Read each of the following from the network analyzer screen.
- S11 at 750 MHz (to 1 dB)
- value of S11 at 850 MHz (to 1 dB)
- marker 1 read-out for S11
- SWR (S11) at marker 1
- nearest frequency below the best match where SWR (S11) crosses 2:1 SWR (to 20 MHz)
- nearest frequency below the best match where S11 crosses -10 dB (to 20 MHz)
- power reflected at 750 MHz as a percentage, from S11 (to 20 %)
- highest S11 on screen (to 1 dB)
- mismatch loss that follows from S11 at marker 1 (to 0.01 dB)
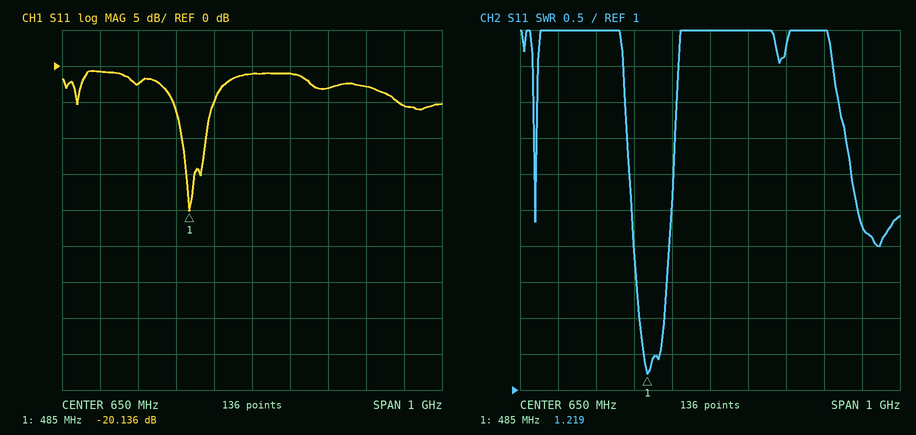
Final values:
-1 dB
-3 dB
-20.136 dB
1.219
460 MHz
460 MHz
80 %
-1 dB
0.04 dB
